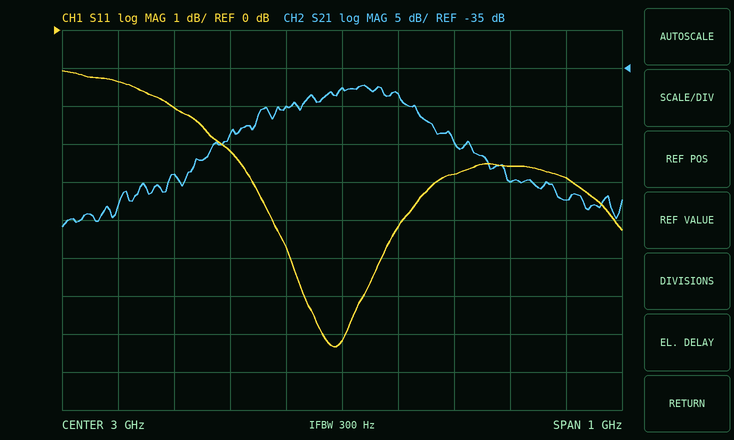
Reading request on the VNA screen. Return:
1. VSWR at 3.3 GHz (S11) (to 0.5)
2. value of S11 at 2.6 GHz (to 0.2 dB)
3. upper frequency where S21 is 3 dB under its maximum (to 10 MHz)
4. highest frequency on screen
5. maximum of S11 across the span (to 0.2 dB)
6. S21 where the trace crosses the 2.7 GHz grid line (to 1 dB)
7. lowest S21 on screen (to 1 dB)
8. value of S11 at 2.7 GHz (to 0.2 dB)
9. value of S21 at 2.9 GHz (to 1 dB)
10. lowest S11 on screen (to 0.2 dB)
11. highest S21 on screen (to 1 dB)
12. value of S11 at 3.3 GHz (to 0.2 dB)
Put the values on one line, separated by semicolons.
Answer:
5.0; -1.4 dB; 3.13 GHz; 3.5 GHz; -1.0 dB; -49 dB; -56 dB; -2.0 dB; -40 dB; -8.4 dB; -37 dB; -3.6 dB
